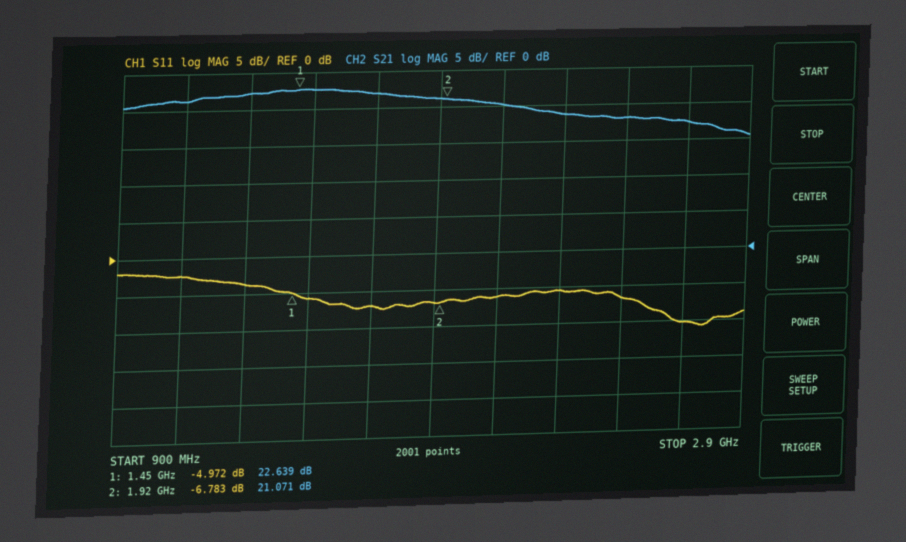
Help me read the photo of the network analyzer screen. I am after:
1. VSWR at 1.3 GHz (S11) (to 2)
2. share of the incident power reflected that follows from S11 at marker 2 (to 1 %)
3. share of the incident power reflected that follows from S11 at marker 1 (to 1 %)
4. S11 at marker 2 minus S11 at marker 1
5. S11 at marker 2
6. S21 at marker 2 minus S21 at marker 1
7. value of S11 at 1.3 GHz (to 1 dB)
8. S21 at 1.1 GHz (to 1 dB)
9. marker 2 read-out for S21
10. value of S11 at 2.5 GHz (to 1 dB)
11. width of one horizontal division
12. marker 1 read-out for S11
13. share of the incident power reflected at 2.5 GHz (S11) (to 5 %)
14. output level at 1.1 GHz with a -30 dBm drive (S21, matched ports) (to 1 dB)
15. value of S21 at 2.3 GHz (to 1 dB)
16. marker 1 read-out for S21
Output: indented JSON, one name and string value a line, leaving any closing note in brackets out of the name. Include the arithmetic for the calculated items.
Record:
{
  "VSWR at 1.3 GHz (S11)": "|Γ| = 10^(-4/20) = 0.6310; VSWR = (1 + 0.6310)/(1 − 0.6310) ≈ 4",
  "share of the incident power reflected that follows from S11 at marker 2": "10^(-6.783/10) ≈ 21 %",
  "share of the incident power reflected that follows from S11 at marker 1": "10^(-4.972/10) ≈ 32 %",
  "S11 at marker 2 minus S11 at marker 1": "-6.783 − (-4.972) = -1.811 dB",
  "S11 at marker 2": "-6.783 dB",
  "S21 at marker 2 minus S21 at marker 1": "21.071 − (22.639) = -1.568 dB",
  "value of S11 at 1.3 GHz": "-4 dB",
  "S21 at 1.1 GHz": "21 dB",
  "marker 2 read-out for S21": "21.071 dB",
  "value of S11 at 2.5 GHz": "-7 dB",
  "width of one horizontal division": "200 MHz",
  "marker 1 read-out for S11": "-4.972 dB",
  "share of the incident power reflected at 2.5 GHz (S11)": "10^(-7/10) ≈ 20 %",
  "output level at 1.1 GHz with a -30 dBm drive (S21, matched ports)": "-30 dBm + (21 dB) = -9 dBm",
  "value of S21 at 2.3 GHz": "19 dB",
  "marker 1 read-out for S21": "22.639 dB"
}
